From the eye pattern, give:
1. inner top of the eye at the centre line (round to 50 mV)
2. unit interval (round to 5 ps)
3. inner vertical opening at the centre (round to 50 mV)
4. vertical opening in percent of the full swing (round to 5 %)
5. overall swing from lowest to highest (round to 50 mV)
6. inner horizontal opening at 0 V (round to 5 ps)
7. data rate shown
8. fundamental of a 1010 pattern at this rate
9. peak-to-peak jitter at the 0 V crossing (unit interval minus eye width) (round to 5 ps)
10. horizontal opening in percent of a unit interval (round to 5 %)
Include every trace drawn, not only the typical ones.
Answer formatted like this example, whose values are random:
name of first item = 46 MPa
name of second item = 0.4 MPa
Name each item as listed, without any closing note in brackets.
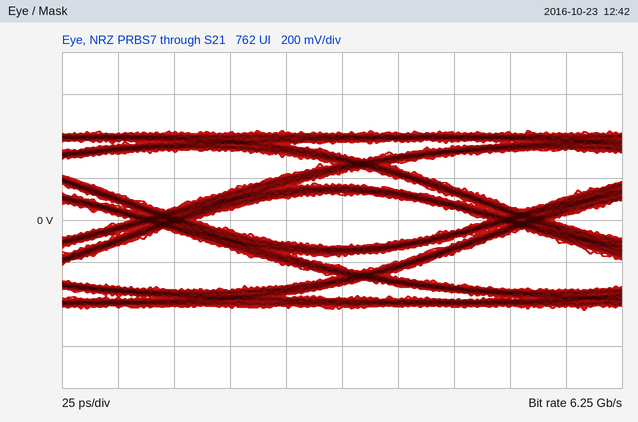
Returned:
inner top of the eye at the centre line = 100 mV
unit interval = 160 ps
inner vertical opening at the centre = 250 mV
vertical opening in percent of the full swing = 30 %
overall swing from lowest to highest = 850 mV
inner horizontal opening at 0 V = 130 ps
data rate shown = 6.25 Gb/s
fundamental of a 1010 pattern at this rate = 3.125 GHz
peak-to-peak jitter at the 0 V crossing (unit interval minus eye width) = 30 ps
horizontal opening in percent of a unit interval = 80 %
